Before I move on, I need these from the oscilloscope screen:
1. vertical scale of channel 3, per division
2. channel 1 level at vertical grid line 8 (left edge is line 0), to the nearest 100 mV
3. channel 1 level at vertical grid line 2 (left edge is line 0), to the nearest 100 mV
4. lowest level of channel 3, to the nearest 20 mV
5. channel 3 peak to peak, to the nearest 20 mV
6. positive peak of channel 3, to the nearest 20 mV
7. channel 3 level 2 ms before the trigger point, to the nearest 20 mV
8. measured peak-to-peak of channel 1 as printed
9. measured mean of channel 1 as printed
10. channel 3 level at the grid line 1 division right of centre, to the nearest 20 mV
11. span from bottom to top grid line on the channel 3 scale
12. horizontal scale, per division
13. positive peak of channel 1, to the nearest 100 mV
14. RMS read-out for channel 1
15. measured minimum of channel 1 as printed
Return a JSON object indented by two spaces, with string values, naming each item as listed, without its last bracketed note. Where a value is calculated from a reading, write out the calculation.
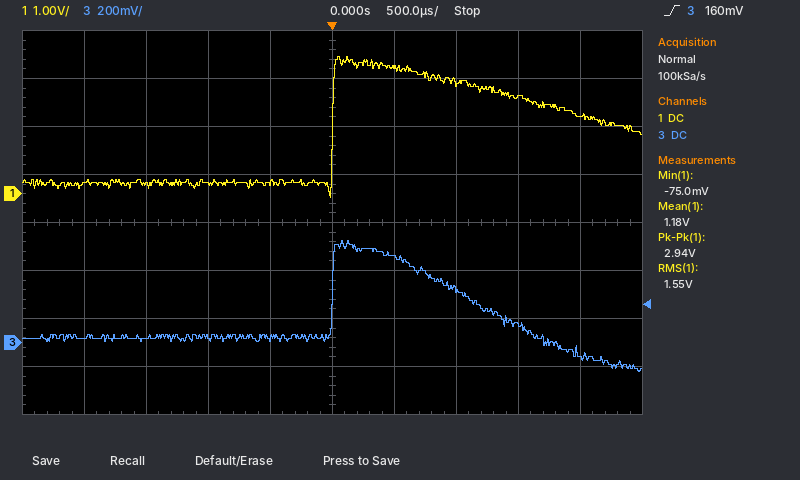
{
  "vertical scale of channel 3, per division": "200 mV",
  "channel 1 level at vertical grid line 8 (left edge is line 0), to the nearest 100 mV": "2.0 V",
  "channel 1 level at vertical grid line 2 (left edge is line 0), to the nearest 100 mV": "200 mV",
  "lowest level of channel 3, to the nearest 20 mV": "-120 mV",
  "channel 3 peak to peak, to the nearest 20 mV": "420 mV − (-120 mV) = 540 mV",
  "positive peak of channel 3, to the nearest 20 mV": "420 mV",
  "channel 3 level 2 ms before the trigger point, to the nearest 20 mV": "20 mV",
  "measured peak-to-peak of channel 1 as printed": "2.94 V",
  "measured mean of channel 1 as printed": "1.18 V",
  "channel 3 level at the grid line 1 division right of centre, to the nearest 20 mV": "360 mV",
  "span from bottom to top grid line on the channel 3 scale": "1.6 V",
  "horizontal scale, per division": "500 µs",
  "positive peak of channel 1, to the nearest 100 mV": "2.9 V",
  "RMS read-out for channel 1": "1.55 V",
  "measured minimum of channel 1 as printed": "-75.0 mV"
}
